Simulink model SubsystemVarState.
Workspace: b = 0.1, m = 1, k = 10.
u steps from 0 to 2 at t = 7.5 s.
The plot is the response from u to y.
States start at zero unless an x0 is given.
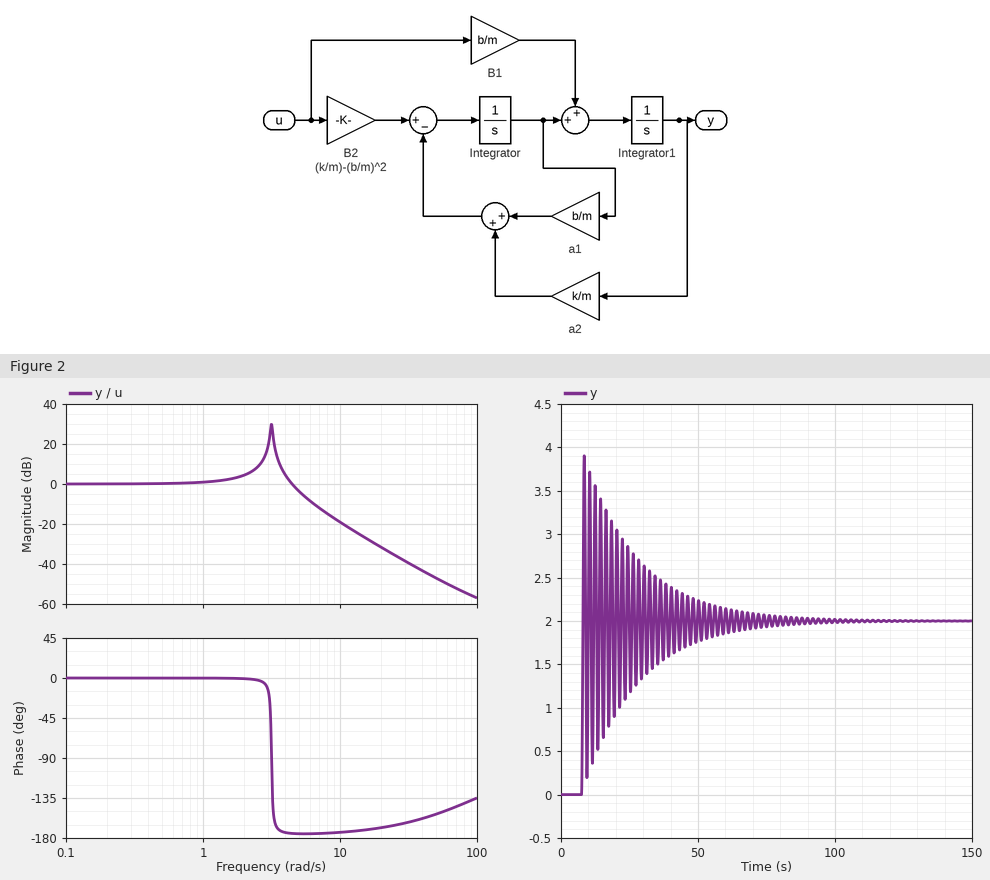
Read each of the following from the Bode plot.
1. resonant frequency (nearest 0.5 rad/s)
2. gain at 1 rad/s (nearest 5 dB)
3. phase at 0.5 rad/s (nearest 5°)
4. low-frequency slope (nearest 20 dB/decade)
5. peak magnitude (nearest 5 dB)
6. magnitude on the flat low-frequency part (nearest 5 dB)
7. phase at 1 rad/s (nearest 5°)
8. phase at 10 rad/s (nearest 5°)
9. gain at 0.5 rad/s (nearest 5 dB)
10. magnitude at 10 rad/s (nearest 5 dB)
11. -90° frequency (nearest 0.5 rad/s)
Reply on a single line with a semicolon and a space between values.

3.0 rad/s; 0 dB; 0°; 0 dB/decade; 30 dB; 0 dB; 0°; -175°; 0 dB; -20 dB; 3.0 rad/s
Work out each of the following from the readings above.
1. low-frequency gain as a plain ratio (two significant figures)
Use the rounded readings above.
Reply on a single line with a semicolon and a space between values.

1.0
